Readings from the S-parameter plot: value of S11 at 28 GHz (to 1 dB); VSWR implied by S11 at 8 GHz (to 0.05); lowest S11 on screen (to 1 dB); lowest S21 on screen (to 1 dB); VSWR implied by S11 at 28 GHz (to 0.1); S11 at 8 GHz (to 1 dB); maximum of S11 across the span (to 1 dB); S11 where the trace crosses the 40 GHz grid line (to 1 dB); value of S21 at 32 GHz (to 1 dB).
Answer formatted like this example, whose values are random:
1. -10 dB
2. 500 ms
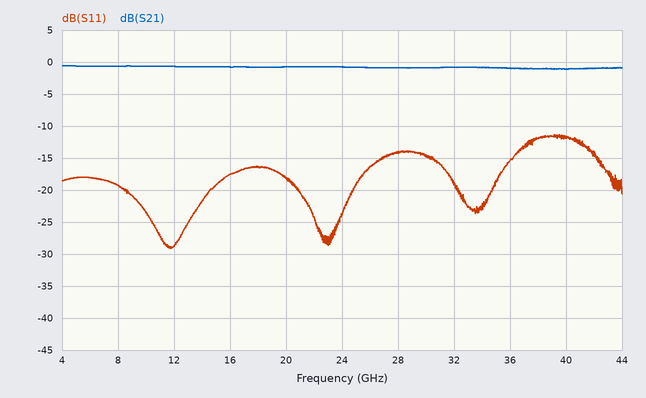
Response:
1. -14 dB
2. 1.25
3. -29 dB
4. -1 dB
5. 1.5
6. -19 dB
7. -11 dB
8. -12 dB
9. -1 dB
